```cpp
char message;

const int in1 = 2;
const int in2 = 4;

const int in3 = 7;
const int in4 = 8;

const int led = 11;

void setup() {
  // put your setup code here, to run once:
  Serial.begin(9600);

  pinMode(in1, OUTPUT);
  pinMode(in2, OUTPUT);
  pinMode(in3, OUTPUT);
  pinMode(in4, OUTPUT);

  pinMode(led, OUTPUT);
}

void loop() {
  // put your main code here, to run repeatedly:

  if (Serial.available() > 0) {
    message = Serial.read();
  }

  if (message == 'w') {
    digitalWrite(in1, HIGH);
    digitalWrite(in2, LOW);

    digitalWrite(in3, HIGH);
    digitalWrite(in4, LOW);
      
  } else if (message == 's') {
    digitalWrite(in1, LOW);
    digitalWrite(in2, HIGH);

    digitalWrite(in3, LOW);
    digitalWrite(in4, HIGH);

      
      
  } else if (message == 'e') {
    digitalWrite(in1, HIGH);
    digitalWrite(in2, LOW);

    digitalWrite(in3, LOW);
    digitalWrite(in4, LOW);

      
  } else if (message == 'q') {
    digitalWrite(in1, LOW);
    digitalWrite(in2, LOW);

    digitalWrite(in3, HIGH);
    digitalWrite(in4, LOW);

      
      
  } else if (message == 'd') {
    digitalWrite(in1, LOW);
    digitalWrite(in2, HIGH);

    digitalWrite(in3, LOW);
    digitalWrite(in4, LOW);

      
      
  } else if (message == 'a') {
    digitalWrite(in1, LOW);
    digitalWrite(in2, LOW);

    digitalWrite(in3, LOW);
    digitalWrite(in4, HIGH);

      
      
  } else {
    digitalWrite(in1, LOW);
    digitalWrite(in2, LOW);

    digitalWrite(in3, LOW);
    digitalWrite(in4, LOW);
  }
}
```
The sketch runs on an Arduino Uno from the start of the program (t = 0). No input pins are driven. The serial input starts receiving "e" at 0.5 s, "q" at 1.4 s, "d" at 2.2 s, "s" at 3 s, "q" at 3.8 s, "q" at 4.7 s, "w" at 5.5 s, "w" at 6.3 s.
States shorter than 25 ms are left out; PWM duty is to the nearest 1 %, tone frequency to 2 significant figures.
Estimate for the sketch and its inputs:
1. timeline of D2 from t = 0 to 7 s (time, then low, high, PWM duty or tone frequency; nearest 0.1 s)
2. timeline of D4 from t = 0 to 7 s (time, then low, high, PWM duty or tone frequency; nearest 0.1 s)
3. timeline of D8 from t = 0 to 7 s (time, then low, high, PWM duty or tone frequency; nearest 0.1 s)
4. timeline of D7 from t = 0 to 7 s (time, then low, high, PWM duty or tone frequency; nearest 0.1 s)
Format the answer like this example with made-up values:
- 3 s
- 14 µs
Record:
- 0 s low; 0.5 s high; 1.4 s low; 5.5 s high
- 0 s low; 2.2 s high; 3.8 s low
- 0 s low; 3 s high; 3.8 s low
- 0 s low; 1.4 s high; 2.2 s low; 3.8 s high
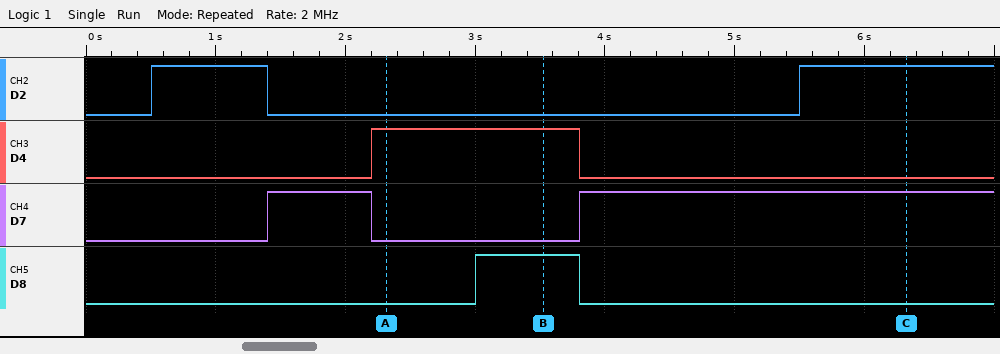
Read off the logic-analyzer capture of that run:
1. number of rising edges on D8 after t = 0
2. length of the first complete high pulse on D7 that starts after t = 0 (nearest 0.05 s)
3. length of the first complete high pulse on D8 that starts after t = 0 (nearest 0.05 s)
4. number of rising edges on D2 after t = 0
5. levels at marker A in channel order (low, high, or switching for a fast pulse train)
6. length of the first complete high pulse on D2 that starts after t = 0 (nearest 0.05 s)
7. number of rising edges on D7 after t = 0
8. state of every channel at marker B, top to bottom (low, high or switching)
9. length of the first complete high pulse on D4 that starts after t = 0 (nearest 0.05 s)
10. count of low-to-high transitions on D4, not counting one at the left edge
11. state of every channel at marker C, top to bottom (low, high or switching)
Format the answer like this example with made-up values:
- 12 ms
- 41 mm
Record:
- 1
- 0.80 s
- 0.80 s
- 2
- D2 low, D4 high, D7 low, D8 low
- 0.90 s
- 2
- D2 low, D4 high, D7 low, D8 high
- 1.60 s
- 1
- D2 high, D4 low, D7 high, D8 low
